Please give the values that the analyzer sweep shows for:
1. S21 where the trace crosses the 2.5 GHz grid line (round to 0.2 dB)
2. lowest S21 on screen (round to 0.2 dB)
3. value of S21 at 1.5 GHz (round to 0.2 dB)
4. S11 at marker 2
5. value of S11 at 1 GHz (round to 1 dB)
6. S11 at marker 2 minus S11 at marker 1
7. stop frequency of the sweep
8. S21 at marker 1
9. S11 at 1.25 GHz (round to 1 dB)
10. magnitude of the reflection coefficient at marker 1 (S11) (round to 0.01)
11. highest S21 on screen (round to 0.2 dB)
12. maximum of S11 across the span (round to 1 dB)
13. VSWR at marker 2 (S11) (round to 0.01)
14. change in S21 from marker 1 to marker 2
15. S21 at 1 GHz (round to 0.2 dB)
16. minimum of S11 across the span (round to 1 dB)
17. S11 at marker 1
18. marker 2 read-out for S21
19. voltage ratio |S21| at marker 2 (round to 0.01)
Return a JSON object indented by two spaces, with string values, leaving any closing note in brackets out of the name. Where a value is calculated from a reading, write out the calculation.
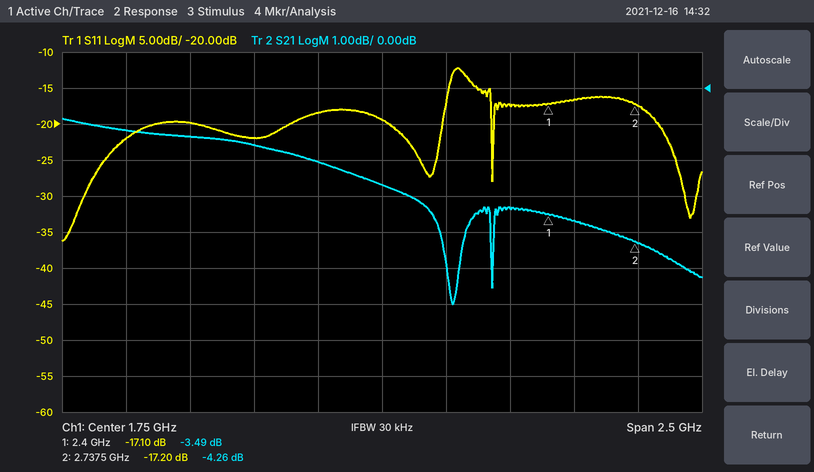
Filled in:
{
  "S21 where the trace crosses the 2.5 GHz grid line": "-3.6 dB",
  "lowest S21 on screen": "-6.0 dB",
  "value of S21 at 1.5 GHz": "-2.0 dB",
  "S11 at marker 2": "-17.20 dB",
  "value of S11 at 1 GHz": "-20 dB",
  "S11 at marker 2 minus S11 at marker 1": "-17.2 − (-17.1) = -0.10 dB",
  "stop frequency of the sweep": "3 GHz",
  "S21 at marker 1": "-3.49 dB",
  "S11 at 1.25 GHz": "-22 dB",
  "magnitude of the reflection coefficient at marker 1 (S11)": "10^(-17.1/20) ≈ 0.14",
  "highest S21 on screen": "-0.8 dB",
  "maximum of S11 across the span": "-12 dB",
  "VSWR at marker 2 (S11)": "(1 + 0.1380)/(1 − 0.1380) ≈ 1.32",
  "change in S21 from marker 1 to marker 2": "-4.26 − (-3.49) = -0.77 dB",
  "S21 at 1 GHz": "-1.4 dB",
  "minimum of S11 across the span": "-36 dB",
  "S11 at marker 1": "-17.10 dB",
  "marker 2 read-out for S21": "-4.26 dB",
  "voltage ratio |S21| at marker 2": "10^(-4.26/20) ≈ 0.61"
}
